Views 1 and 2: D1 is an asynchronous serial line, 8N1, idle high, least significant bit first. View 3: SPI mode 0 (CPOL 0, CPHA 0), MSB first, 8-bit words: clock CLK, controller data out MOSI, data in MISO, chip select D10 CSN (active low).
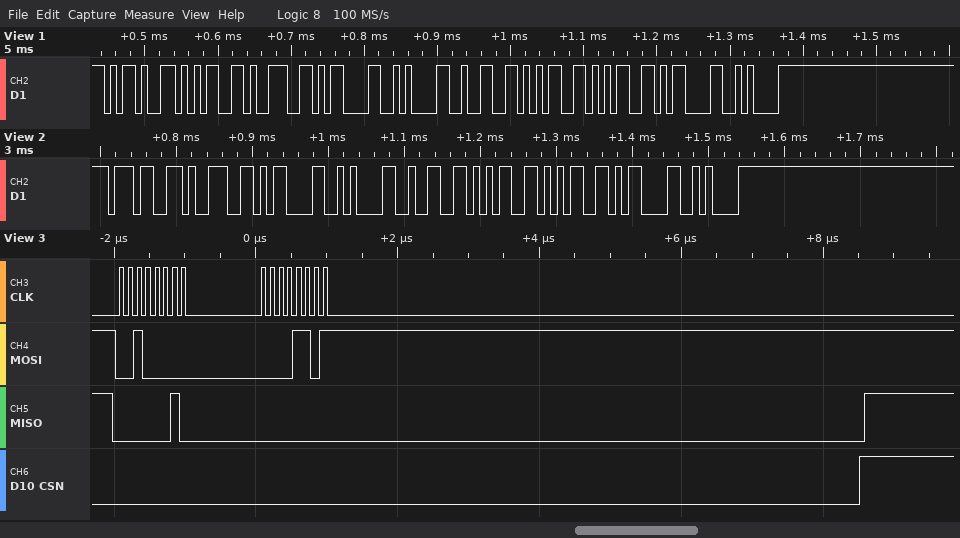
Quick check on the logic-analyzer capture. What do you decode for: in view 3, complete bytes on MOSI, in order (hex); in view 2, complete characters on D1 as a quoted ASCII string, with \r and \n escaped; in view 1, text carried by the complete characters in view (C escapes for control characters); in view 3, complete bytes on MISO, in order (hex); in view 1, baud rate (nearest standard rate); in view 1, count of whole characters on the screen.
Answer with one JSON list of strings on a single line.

["20 0D", "\"79\\r\\n255\\r\\n\"", "\"-59\\r\\n255\\r\\n\"", "02 00", "115200 baud", "10"]
